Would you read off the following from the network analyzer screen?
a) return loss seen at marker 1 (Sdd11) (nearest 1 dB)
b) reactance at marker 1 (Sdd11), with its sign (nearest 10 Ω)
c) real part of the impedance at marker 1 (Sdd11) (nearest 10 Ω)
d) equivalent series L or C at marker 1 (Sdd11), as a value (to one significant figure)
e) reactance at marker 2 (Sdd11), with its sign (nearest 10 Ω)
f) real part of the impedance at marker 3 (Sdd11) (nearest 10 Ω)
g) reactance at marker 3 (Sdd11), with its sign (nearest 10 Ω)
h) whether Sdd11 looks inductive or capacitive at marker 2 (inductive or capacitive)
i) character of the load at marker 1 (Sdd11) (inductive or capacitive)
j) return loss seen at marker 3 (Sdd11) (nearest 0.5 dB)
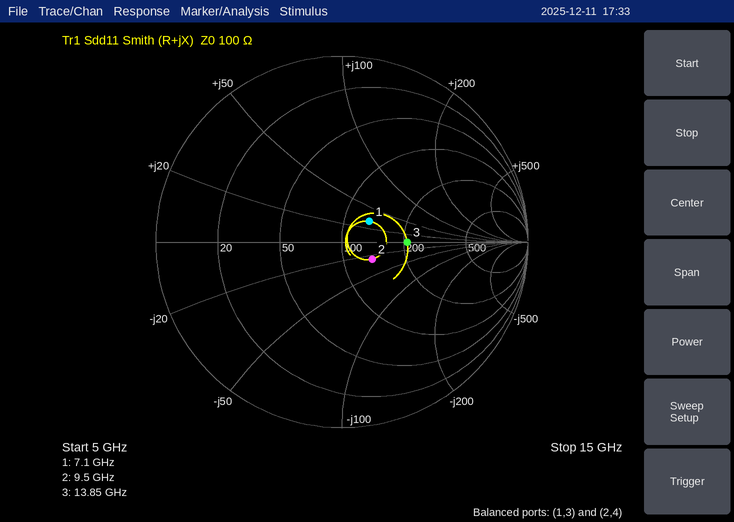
15 dB
+30 Ω
130 Ω
700 pH
-30 Ω
210 Ω
0 Ω
capacitive
inductive
9.0 dB
